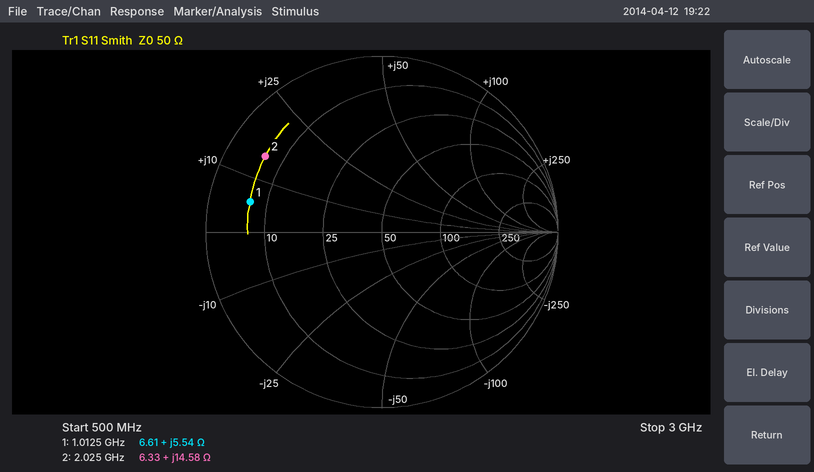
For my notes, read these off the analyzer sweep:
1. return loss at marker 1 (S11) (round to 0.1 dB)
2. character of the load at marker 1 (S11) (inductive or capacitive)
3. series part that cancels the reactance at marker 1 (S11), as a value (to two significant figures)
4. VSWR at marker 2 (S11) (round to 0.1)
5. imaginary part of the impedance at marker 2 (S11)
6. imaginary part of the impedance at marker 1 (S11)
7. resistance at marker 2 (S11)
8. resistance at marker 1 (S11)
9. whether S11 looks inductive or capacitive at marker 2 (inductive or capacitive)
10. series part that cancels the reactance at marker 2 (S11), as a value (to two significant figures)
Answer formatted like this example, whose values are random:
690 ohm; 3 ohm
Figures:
2.3 dB; inductive; 28 pF; 8.6; +14.58 Ω; +5.54 Ω; 6.33 Ω; 6.61 Ω; inductive; 5.4 pF
